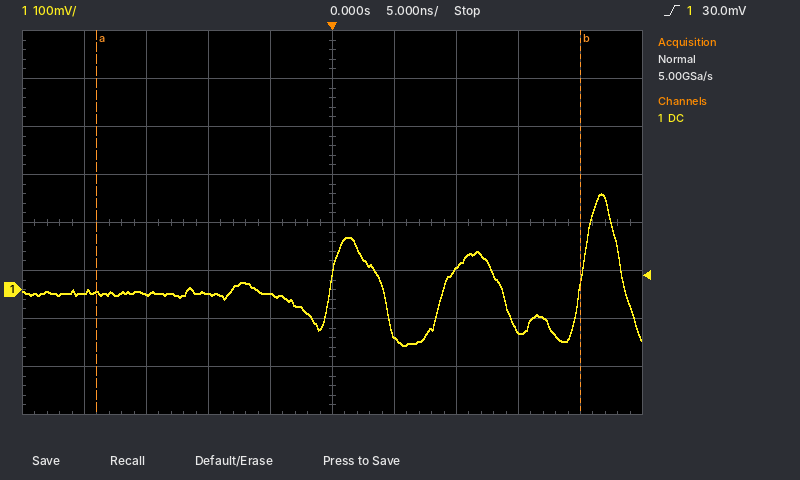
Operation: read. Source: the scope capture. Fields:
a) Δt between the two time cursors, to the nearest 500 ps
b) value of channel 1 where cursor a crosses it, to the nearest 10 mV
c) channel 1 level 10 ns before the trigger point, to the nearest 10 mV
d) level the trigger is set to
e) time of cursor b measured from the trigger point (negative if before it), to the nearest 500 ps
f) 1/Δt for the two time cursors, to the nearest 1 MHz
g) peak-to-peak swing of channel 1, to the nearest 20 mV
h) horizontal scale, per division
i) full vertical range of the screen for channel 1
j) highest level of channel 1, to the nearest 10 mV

39.0 ns
-10 mV
-10 mV
30.0 mV
+20.0 ns
26 MHz
320 mV
5 ns
800 mV
200 mV
